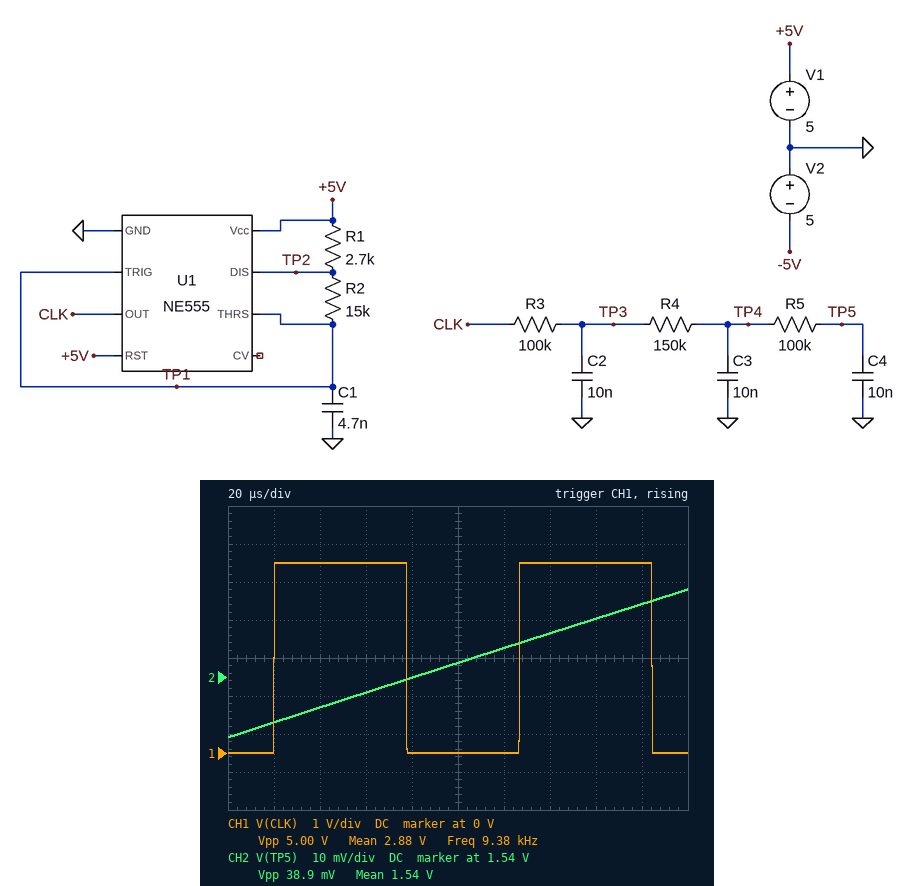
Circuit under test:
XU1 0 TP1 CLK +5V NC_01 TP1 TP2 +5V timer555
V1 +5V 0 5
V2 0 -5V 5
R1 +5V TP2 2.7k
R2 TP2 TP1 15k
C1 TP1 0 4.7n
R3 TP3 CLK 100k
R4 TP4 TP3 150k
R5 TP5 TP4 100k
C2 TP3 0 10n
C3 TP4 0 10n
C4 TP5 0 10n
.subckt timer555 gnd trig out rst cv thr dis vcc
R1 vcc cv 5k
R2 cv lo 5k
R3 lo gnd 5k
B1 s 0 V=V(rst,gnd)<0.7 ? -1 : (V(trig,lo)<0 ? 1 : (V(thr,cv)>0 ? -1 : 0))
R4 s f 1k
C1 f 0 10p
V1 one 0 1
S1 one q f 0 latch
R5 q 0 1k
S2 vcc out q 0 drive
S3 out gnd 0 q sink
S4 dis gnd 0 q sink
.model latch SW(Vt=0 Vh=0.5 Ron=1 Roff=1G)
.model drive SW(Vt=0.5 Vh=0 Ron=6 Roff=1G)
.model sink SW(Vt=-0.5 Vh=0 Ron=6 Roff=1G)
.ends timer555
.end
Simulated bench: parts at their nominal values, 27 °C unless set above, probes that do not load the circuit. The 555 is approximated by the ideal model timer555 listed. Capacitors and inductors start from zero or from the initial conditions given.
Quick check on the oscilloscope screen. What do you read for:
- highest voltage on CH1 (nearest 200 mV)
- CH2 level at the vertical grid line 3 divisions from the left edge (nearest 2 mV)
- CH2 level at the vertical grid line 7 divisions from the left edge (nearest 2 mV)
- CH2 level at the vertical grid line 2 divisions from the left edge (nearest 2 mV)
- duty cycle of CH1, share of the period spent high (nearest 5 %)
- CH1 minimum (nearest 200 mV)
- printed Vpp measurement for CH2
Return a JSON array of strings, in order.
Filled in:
["5.0 V", "1.536 V", "1.552 V", "1.532 V", "55 %", "0 V", "38.9 mV"]
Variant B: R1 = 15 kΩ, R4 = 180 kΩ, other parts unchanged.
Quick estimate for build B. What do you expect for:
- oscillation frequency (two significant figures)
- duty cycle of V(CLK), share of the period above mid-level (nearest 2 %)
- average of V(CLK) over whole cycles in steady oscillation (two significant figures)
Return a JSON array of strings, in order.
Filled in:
["6.8 kHz", "66 %", "3.3 V"]
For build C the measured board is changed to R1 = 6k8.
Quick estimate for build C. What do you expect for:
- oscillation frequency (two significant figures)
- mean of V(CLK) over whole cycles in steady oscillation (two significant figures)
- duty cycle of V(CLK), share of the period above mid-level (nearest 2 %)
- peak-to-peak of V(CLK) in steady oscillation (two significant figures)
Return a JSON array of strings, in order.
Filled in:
["8.3 kHz", "3.0 V", "60 %", "5.0 V"]
